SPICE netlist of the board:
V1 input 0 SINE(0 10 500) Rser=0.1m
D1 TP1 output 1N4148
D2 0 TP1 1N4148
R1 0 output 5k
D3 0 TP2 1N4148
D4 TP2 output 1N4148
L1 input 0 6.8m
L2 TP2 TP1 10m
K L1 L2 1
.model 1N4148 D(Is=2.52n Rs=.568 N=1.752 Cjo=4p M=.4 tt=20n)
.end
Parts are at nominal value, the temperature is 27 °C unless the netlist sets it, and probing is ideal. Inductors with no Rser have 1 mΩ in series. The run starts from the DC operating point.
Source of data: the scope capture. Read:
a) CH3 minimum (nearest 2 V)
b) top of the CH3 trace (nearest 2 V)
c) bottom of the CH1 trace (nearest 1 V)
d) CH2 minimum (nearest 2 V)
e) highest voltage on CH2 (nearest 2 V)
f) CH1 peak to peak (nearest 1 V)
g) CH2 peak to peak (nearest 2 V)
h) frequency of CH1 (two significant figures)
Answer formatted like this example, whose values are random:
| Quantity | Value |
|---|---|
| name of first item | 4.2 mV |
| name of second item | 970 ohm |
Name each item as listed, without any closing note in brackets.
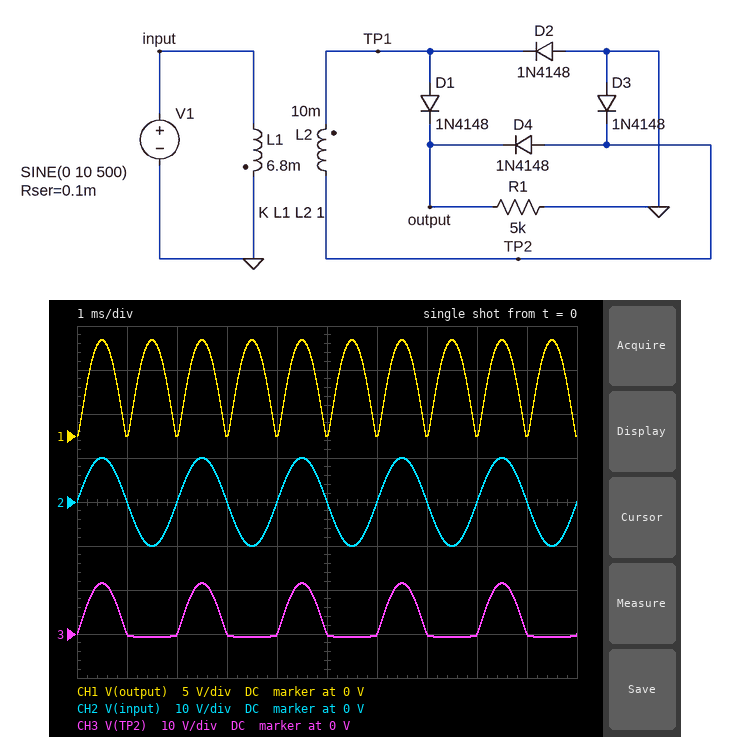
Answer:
| Quantity | Value |
|---|---|
| CH3 minimum | 0 V |
| top of the CH3 trace | 12 V |
| bottom of the CH1 trace | 0 V |
| CH2 minimum | -10 V |
| highest voltage on CH2 | 10 V |
| CH1 peak to peak | 11 V |
| CH2 peak to peak | 20 V |
| frequency of CH1 | 1.0 kHz |
